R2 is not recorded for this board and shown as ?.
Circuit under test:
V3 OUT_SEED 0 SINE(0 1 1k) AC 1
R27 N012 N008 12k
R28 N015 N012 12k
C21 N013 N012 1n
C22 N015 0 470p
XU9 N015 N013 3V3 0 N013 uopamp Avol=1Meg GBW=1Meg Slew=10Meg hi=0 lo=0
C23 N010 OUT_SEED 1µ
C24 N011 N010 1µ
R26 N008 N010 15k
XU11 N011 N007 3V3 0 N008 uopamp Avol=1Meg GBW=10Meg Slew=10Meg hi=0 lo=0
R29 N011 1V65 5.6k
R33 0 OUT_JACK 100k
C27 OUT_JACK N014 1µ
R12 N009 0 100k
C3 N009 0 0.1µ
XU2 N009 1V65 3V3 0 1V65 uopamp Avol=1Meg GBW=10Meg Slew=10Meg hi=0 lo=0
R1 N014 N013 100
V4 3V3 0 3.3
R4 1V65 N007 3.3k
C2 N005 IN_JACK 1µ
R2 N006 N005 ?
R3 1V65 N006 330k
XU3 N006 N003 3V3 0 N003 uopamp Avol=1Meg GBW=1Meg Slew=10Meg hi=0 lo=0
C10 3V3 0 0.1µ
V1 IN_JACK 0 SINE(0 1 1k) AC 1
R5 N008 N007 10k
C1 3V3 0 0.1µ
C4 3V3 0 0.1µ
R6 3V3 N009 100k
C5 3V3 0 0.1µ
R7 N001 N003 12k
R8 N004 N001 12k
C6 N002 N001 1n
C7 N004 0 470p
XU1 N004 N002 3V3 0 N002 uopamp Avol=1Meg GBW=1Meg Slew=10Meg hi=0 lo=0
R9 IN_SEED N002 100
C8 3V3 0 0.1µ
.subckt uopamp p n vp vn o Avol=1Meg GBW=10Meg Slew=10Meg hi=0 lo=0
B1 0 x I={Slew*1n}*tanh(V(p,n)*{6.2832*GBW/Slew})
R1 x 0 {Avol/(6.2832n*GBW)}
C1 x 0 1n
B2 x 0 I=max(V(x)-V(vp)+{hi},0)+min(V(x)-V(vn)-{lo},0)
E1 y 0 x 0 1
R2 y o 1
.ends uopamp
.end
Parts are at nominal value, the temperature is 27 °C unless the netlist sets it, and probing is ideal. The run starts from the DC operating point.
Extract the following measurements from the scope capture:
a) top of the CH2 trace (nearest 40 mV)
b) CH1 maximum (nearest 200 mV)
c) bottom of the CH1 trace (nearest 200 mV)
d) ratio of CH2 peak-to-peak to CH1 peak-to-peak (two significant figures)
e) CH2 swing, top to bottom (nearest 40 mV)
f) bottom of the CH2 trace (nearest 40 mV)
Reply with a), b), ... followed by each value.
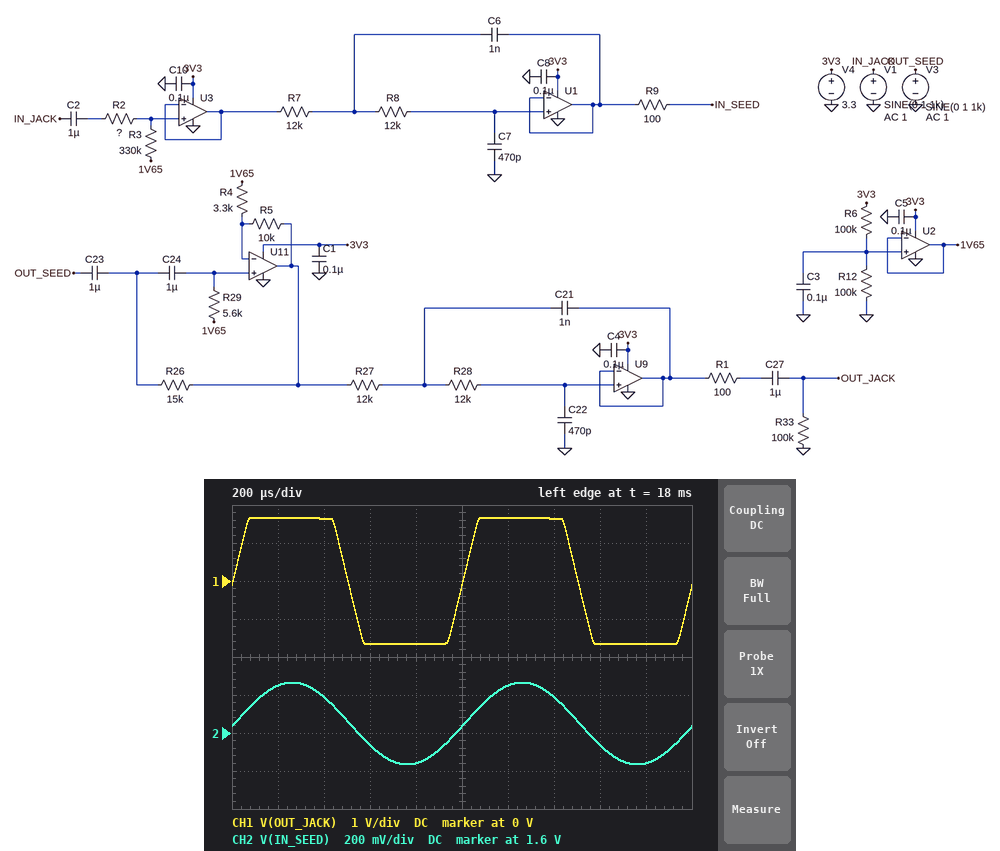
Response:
a) 1.88 V
b) 1.6 V
c) -1.6 V
d) 0.13
e) 440 mV
f) 1.44 V
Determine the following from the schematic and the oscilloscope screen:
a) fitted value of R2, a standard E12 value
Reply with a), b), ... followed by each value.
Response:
a) 1.2 MΩ
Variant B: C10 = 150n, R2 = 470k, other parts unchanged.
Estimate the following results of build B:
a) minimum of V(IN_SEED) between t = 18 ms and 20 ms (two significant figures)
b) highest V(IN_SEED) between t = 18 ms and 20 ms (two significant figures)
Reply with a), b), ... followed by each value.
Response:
a) 1.2 V
b) 2.1 V
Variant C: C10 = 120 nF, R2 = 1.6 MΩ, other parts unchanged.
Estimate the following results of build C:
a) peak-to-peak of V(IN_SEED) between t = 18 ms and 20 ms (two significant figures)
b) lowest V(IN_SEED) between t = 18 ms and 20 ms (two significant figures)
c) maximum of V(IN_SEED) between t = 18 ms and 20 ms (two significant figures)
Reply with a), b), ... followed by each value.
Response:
a) 340 mV
b) 1.5 V
c) 1.8 V
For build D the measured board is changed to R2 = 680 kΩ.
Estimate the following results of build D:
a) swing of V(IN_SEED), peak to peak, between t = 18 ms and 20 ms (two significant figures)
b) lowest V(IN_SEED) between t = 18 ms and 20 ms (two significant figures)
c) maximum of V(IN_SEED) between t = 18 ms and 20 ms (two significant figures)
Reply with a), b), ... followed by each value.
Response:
a) 650 mV
b) 1.3 V
c) 2.0 V
